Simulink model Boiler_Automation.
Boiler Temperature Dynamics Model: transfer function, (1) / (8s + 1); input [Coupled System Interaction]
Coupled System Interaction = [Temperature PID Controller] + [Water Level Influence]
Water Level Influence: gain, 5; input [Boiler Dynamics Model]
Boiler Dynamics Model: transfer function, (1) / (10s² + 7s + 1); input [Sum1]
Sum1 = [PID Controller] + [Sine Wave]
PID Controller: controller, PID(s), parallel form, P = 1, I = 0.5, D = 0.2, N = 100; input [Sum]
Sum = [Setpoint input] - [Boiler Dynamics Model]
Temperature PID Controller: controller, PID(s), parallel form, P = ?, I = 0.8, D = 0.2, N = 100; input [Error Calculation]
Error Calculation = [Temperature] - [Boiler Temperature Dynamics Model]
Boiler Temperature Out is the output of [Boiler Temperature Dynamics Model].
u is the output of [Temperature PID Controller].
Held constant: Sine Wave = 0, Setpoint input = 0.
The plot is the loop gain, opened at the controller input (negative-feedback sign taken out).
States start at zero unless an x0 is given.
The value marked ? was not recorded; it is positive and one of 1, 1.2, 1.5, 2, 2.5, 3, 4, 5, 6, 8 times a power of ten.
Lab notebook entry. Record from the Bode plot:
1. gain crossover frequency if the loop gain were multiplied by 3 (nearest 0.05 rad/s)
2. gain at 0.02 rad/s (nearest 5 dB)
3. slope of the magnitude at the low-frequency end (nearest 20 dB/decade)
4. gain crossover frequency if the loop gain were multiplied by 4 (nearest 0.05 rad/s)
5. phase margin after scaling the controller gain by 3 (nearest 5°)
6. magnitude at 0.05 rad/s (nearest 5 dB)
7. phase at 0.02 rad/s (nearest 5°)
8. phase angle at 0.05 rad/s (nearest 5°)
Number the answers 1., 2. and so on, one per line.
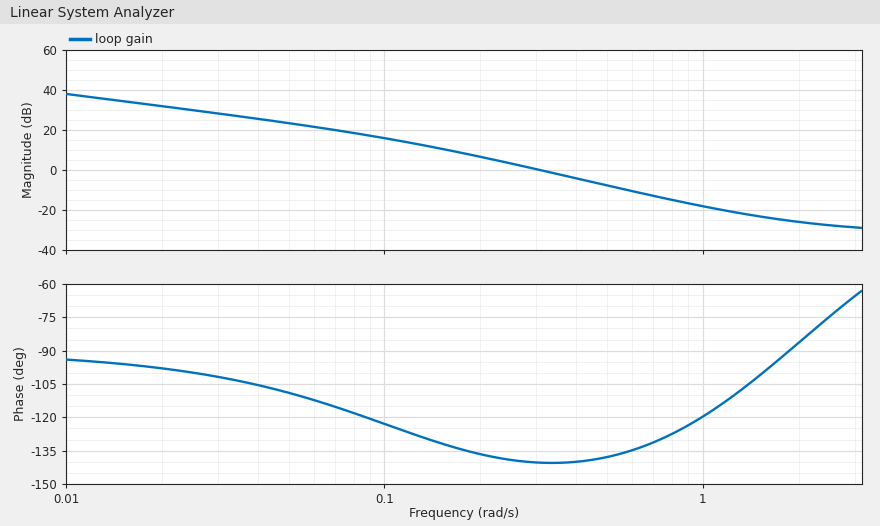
1. 0.55 rad/s
2. 30 dB
3. -20 dB/decade
4. 0.65 rad/s
5. 45°
6. 25 dB
7. -100°
8. -110°
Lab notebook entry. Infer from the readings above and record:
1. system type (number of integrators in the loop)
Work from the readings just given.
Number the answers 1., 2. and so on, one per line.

1. 1
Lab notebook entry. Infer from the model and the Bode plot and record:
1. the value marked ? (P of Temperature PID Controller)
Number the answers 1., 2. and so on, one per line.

1. 0.8
